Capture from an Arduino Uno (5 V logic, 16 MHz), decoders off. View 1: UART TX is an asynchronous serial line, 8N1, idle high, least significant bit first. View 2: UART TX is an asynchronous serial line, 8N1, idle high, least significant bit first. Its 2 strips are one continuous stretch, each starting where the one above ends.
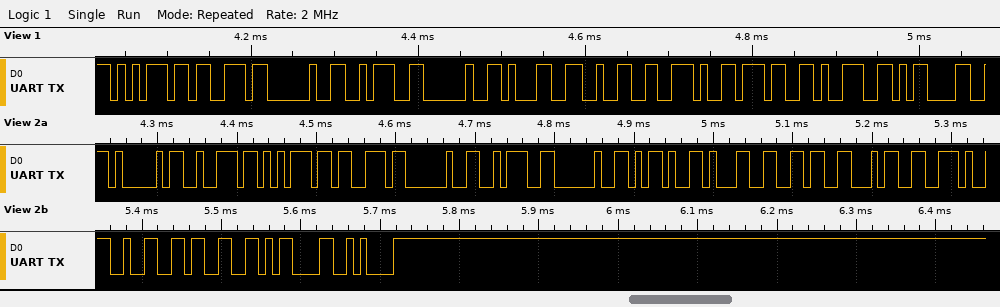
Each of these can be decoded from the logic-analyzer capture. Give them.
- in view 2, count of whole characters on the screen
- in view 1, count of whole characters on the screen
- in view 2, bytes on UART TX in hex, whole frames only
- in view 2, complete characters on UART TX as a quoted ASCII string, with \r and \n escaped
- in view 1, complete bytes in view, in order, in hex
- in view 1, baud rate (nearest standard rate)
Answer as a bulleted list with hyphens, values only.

- 16
- 11
- 41 72 75 73 20 3A 20 2D 31 36 34 2E 32 33 0D 0A
- "Arus : -164.23\r\n"
- 75 73 20 3A 20 31 32 2E 37 39 0D
- 115200 baud
